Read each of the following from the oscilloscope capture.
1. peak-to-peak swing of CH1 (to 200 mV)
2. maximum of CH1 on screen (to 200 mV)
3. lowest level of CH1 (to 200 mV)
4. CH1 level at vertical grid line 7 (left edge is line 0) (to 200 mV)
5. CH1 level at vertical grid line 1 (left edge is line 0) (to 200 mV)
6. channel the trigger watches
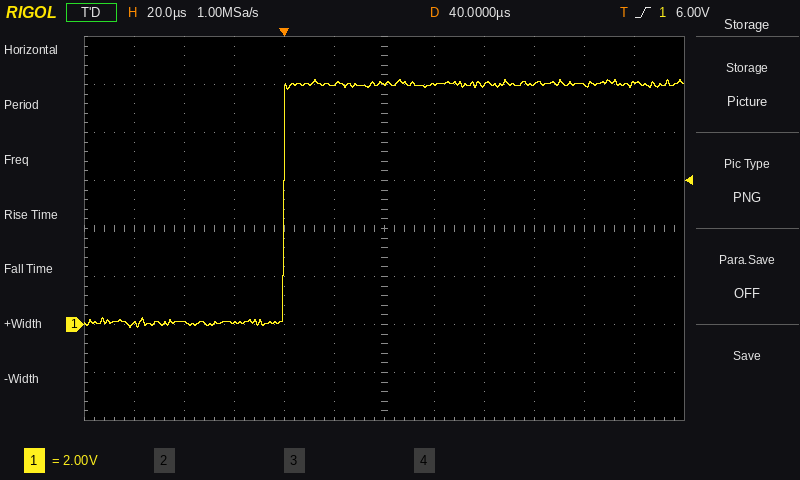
10.4 V
10.2 V
-200 mV
10.0 V
0.0 V
CH1
